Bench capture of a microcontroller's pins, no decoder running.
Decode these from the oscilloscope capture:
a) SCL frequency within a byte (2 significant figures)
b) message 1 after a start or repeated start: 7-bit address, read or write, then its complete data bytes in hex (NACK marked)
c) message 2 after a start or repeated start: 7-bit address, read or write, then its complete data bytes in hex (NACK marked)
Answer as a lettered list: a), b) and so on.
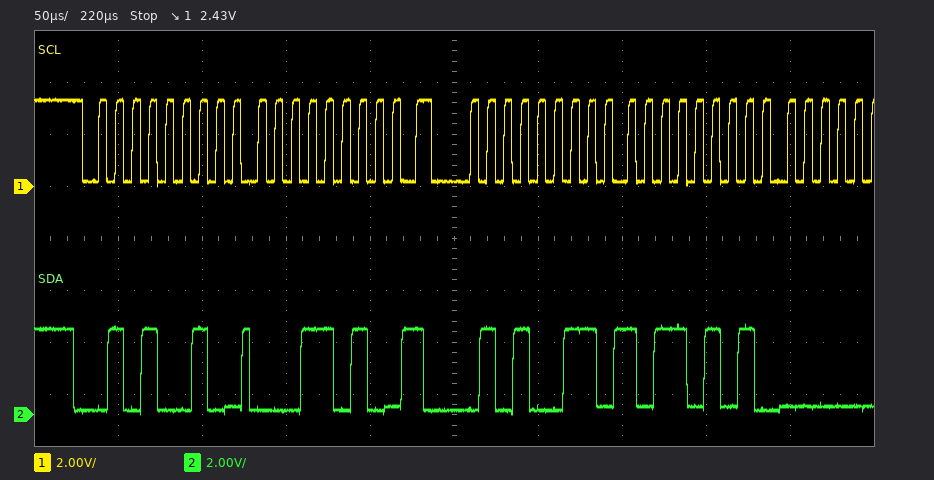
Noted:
a) 100 kHz
b) 0x29 write: 1A
c) 0x29 read: B5
